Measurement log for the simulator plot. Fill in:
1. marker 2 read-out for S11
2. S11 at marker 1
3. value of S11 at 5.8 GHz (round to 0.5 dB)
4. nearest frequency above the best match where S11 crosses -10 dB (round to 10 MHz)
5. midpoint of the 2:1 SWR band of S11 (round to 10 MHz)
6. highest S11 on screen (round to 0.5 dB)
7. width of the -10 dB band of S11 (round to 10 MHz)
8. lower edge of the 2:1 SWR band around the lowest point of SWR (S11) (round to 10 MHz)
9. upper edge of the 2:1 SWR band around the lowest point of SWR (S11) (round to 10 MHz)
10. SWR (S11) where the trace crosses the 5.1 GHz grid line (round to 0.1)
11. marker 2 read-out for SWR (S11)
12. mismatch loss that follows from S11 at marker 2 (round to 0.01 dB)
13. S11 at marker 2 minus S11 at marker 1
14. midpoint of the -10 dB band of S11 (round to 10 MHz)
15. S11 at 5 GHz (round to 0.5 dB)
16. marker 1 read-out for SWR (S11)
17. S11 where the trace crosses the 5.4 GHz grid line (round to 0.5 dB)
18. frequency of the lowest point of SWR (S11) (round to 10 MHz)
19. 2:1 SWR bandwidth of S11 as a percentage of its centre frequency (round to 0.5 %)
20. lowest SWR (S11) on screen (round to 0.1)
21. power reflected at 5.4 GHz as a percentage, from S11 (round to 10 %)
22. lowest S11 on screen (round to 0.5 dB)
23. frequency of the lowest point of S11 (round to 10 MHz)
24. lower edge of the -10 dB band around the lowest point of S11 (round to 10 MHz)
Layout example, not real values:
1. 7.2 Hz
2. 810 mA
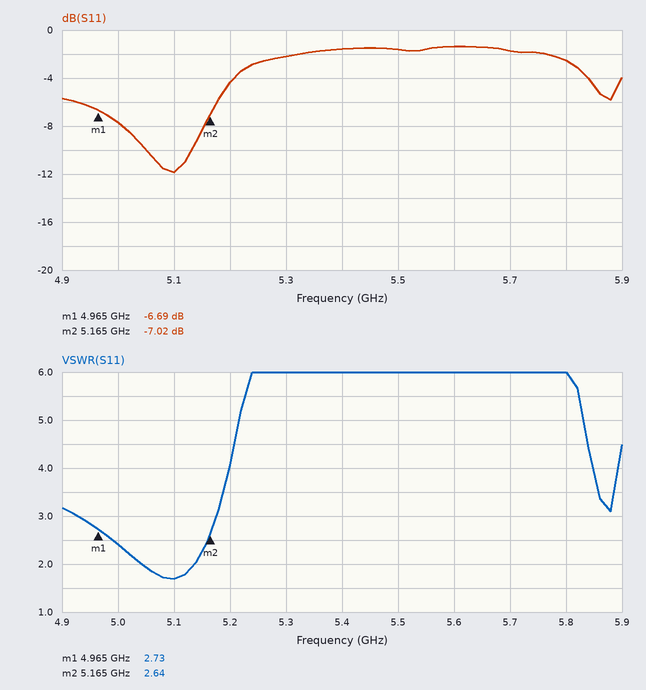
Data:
1. -7.02 dB
2. -6.69 dB
3. -2.5 dB
4. 5.13 GHz
5. 5.09 GHz
6. -1.5 dB
7. 80 MHz
8. 5.04 GHz
9. 5.14 GHz
10. 1.7
11. 2.64
12. 0.96 dB
13. -0.33 dB
14. 5.09 GHz
15. -7.5 dB
16. 2.73
17. -1.5 dB
18. 5.10 GHz
19. 2.0 %
20. 1.7
21. 70 %
22. -12.0 dB
23. 5.10 GHz
24. 5.05 GHz
